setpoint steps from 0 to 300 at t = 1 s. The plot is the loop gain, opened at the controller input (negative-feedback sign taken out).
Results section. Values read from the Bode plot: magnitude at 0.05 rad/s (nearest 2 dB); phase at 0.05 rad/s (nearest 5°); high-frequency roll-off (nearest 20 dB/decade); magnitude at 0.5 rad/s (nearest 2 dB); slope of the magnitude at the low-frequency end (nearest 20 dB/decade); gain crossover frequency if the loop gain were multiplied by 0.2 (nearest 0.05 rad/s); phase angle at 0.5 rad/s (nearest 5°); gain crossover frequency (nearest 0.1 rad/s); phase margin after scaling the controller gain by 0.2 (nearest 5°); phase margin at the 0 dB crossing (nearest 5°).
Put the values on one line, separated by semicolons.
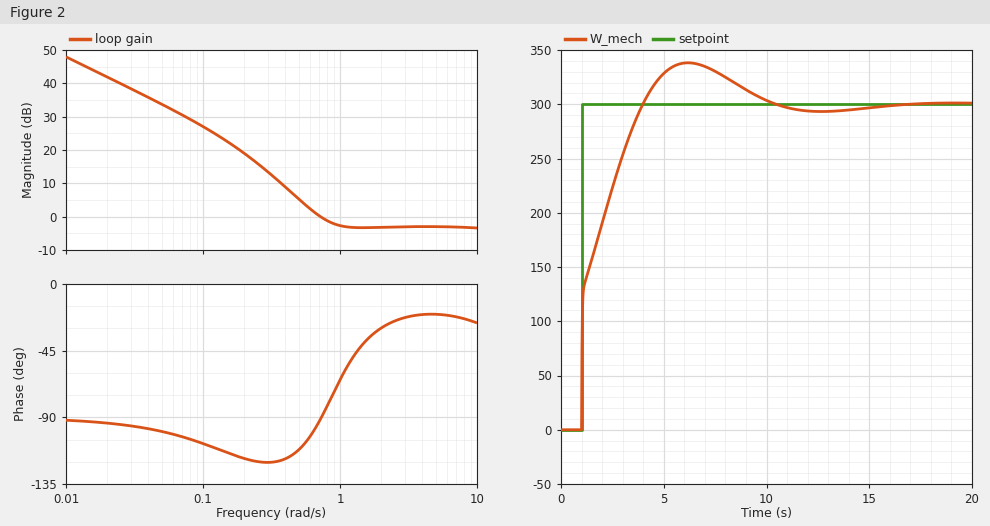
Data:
34 dB; -100°; 0 dB/decade; 6 dB; -20 dB/decade; 0.30 rad/s; -110°; 0.7 rad/s; 60°; 90°
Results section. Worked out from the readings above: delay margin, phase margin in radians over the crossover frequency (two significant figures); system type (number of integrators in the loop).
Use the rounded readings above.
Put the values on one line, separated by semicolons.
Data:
2.2 s; 1
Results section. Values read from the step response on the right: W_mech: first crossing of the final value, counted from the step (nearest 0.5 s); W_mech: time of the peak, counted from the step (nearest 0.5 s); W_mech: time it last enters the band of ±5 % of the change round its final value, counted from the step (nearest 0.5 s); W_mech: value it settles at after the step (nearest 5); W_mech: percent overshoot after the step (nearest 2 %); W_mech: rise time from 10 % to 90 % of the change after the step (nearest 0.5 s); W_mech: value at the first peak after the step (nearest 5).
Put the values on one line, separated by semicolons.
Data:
3.0 s; 5.0 s; 8.0 s; 300; 12 %; 2.5 s; 340
